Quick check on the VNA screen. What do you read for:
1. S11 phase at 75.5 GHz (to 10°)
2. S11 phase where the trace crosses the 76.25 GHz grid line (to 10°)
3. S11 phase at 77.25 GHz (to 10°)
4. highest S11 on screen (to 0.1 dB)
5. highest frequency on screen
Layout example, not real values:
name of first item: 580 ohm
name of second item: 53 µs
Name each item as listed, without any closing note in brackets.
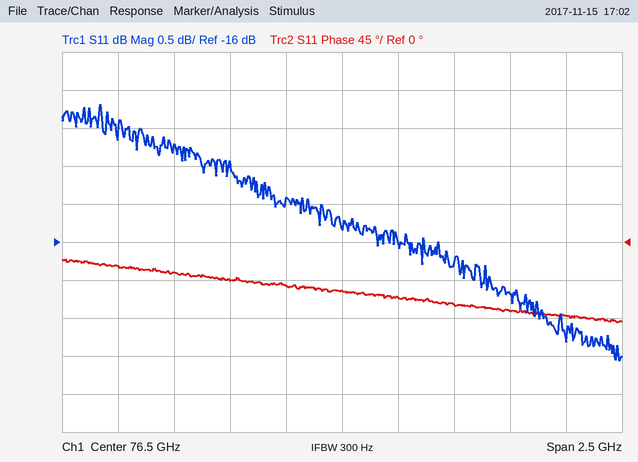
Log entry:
S11 phase at 75.5 GHz: -30°
S11 phase where the trace crosses the 76.25 GHz grid line: -50°
S11 phase at 77.25 GHz: -80°
highest S11 on screen: -14.2 dB
highest frequency on screen: 77.75 GHz
